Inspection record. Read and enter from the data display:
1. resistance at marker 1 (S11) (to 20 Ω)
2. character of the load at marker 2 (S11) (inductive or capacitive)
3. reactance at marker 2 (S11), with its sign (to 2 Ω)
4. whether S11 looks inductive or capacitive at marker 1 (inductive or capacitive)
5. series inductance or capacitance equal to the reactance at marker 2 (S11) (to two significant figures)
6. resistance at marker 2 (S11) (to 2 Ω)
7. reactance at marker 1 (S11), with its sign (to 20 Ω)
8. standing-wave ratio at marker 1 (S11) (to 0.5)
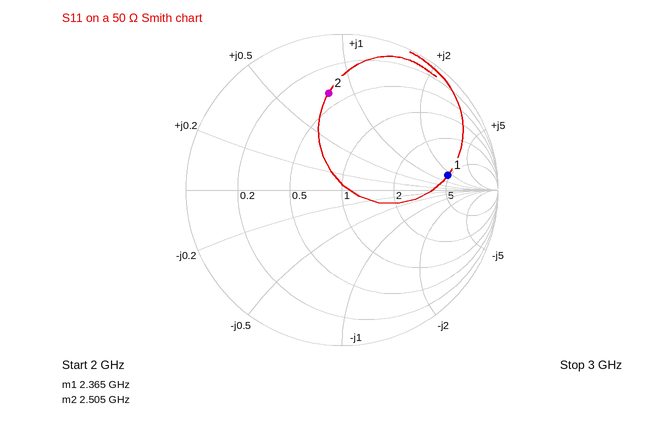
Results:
240 Ω
inductive
+40 Ω
inductive
2.5 nH
20 Ω
+80 Ω
5.5
